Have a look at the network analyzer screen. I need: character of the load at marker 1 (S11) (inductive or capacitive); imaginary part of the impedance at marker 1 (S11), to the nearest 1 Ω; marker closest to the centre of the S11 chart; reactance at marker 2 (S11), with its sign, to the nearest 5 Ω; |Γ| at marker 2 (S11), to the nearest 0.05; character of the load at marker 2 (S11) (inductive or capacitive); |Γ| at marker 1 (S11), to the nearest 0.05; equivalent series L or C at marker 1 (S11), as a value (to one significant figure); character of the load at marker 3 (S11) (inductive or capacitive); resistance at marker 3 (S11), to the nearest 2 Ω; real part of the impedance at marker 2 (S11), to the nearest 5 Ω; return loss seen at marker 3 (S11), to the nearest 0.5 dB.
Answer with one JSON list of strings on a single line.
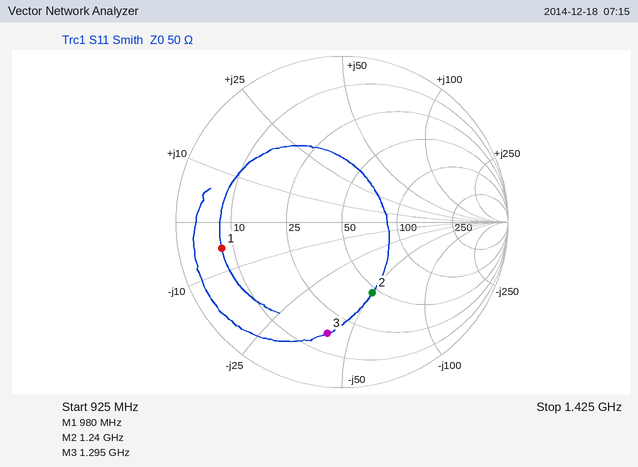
["capacitive", "-5 Ω", "marker 2", "-50 Ω", "0.45", "capacitive", "0.75", "30 pF", "capacitive", "16 Ω", "45 Ω", "3.5 dB"]
